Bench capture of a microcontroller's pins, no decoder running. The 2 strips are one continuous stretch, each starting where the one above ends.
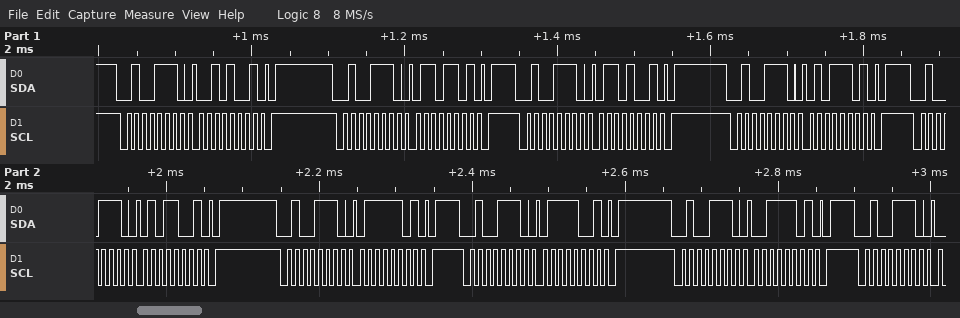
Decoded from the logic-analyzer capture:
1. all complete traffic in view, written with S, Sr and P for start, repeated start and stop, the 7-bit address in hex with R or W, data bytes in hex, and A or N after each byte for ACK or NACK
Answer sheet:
S 27W A 29 A P S 27W A 6D A P S 27W A 69 A P S 27W A 5D A P S 27W A 59 A P S 27W A 7D A P S 27W A 79 A P S 27W A 3D A P S 27W A
